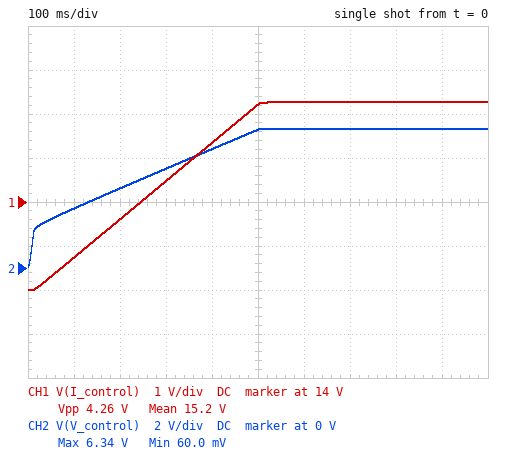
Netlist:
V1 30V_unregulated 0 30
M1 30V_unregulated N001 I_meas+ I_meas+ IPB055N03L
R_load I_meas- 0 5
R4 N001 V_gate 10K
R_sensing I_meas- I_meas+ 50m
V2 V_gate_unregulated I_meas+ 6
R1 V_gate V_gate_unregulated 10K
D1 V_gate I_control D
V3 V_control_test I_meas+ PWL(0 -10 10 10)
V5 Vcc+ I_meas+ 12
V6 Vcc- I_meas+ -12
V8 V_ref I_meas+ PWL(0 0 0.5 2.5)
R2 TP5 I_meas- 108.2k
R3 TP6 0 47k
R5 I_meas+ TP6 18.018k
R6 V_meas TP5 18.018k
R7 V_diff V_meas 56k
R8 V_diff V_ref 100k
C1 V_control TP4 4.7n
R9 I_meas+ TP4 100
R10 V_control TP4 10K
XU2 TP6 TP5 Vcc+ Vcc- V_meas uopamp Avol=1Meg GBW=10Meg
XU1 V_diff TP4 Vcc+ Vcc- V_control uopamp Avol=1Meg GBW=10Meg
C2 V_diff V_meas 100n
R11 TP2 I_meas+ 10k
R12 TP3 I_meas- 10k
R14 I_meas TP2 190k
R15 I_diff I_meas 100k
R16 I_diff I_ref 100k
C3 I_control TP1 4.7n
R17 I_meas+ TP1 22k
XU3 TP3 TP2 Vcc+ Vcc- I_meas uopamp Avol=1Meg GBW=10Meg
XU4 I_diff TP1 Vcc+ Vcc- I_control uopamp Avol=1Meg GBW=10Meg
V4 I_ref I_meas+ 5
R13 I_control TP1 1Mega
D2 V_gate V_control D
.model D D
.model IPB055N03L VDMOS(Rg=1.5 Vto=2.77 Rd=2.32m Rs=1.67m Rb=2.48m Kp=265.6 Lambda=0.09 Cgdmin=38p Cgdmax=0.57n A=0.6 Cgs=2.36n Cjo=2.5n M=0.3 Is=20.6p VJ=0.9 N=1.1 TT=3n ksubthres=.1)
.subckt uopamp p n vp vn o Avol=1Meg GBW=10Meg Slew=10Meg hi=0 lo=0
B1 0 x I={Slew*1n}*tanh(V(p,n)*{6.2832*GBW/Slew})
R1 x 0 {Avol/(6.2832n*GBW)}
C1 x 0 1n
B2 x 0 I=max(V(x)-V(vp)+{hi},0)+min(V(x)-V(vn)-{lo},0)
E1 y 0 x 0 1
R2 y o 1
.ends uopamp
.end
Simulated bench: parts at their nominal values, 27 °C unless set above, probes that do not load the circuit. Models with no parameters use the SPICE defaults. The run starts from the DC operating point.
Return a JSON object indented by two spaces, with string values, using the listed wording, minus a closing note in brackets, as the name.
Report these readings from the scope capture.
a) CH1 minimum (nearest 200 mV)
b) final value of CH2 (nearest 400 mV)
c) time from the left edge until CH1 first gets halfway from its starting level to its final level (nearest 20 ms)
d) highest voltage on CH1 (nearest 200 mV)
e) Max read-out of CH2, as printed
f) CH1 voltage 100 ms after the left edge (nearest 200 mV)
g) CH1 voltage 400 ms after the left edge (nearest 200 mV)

{
  "CH1 minimum": "12.0 V",
  "final value of CH2": "6.4 V",
  "time from the left edge until CH1 first gets halfway from its starting level to its final level": "260 ms",
  "highest voltage on CH1": "16.2 V",
  "Max read-out of CH2, as printed": "6.34 V",
  "CH1 voltage 100 ms after the left edge": "12.8 V",
  "CH1 voltage 400 ms after the left edge": "15.4 V"
}
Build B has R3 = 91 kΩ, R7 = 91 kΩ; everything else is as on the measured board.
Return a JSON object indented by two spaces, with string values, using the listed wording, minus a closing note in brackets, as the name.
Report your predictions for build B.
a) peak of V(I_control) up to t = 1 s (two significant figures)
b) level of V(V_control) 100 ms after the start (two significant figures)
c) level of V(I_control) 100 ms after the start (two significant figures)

{
  "peak of V(I_control) up to t = 1 s": "24 V",
  "level of V(V_control) 100 ms after the start": "4.0 V",
  "level of V(I_control) 100 ms after the start": "14 V"
}
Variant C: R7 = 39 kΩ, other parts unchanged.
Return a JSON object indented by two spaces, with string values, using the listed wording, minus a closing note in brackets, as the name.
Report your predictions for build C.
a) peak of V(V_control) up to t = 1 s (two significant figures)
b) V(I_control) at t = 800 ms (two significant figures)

{
  "peak of V(V_control) up to t = 1 s": "5.0 V",
  "V(I_control) at t = 800 ms": "15 V"
}
